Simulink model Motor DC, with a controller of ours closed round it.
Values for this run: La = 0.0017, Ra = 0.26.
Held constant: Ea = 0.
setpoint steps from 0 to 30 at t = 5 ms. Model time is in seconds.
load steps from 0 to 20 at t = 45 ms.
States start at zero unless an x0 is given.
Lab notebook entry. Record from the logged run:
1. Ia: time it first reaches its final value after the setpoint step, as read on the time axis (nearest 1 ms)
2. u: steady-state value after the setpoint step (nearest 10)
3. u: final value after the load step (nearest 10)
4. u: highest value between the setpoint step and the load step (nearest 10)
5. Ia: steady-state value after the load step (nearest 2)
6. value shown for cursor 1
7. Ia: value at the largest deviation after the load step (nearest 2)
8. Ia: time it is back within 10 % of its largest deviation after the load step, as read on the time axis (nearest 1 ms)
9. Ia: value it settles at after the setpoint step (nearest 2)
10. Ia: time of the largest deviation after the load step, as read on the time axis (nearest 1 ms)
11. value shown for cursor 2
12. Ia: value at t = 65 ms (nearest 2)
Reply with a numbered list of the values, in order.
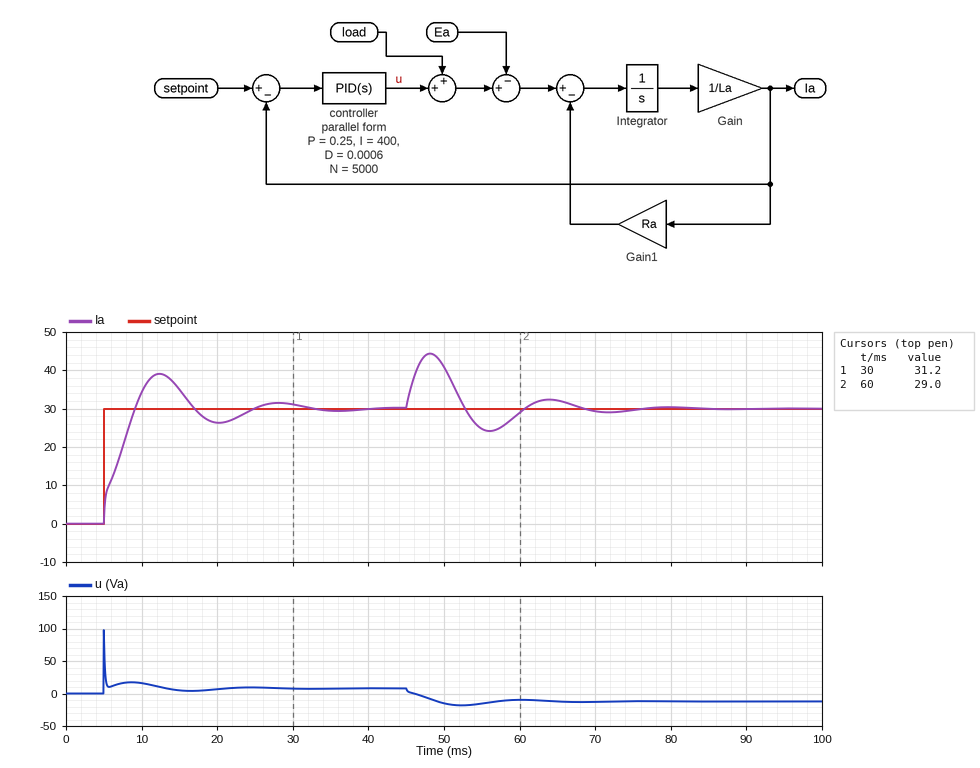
1. 9 ms
2. 10
3. -10
4. 100
5. 30
6. 31.2
7. 44
8. 66 ms
9. 30
10. 48 ms
11. 29.0
12. 32
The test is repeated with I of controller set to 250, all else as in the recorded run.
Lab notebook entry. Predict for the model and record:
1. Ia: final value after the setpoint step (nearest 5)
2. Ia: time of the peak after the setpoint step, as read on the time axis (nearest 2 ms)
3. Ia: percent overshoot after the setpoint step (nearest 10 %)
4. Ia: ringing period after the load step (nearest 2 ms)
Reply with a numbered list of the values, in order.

1. 30
2. 14 ms
3. 20 %
4. 20 ms
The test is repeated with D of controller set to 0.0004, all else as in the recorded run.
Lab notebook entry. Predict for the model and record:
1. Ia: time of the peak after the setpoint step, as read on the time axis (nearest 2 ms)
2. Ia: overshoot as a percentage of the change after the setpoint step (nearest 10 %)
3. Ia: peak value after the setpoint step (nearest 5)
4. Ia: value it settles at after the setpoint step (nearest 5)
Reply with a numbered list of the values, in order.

1. 12 ms
2. 30 %
3. 40
4. 30
